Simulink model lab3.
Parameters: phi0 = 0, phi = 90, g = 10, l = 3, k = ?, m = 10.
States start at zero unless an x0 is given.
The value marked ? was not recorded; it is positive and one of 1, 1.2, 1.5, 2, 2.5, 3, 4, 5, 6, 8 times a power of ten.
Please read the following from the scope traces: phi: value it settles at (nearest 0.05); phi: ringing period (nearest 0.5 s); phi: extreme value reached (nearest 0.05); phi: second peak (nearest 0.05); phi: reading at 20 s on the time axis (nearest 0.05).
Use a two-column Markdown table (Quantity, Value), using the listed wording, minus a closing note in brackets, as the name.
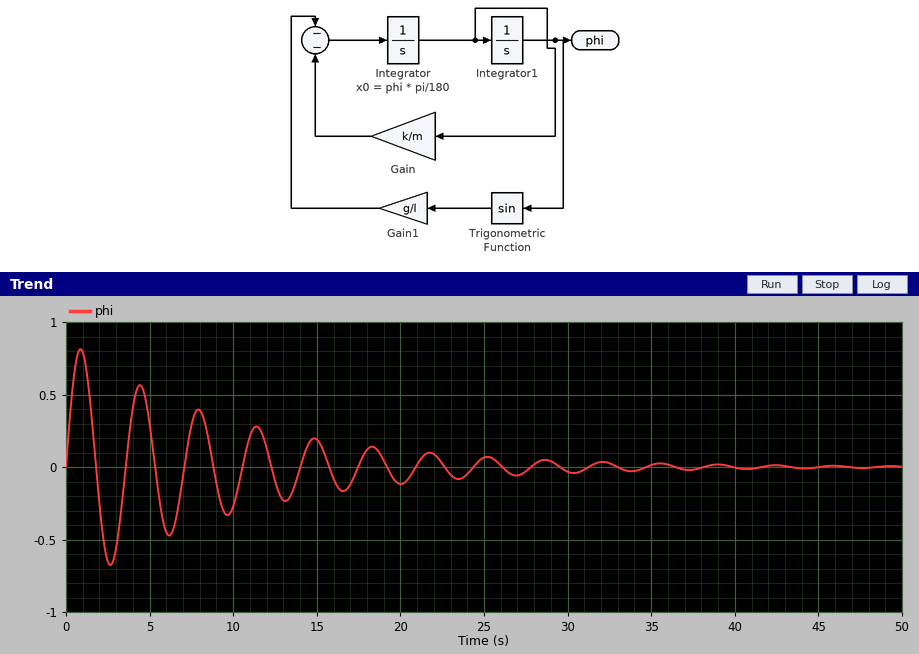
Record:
| Quantity | Value |
|---|---|
| phi: value it settles at | 0.00 |
| phi: ringing period | 3.5 s |
| phi: extreme value reached | 0.80 |
| phi: second peak | 0.55 |
| phi: reading at 20 s on the time axis | -0.10 |
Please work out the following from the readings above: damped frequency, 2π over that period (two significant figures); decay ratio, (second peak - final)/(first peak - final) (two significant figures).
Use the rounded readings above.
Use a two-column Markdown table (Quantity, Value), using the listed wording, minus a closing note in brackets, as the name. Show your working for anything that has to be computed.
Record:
| Quantity | Value |
|---|---|
| damped frequency, 2π over that period | 2π / 3.5 = 1.8 rad/s |
| decay ratio, (second peak - final)/(first peak - final) | (0.55 - 0) / (0.8 - 0) = 0.69 |
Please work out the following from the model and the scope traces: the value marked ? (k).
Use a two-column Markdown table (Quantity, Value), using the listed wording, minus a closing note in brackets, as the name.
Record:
| Quantity | Value |
|---|---|
| the value marked ? | 2 |
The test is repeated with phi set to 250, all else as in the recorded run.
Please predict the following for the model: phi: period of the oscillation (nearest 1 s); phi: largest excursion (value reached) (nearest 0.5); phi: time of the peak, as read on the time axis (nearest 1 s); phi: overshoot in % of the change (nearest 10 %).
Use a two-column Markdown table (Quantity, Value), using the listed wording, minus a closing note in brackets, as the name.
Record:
| Quantity | Value |
|---|---|
| phi: period of the oscillation | 4 s |
| phi: largest excursion (value reached) | 8.5 |
| phi: time of the peak, as read on the time axis | 4 s |
| phi: overshoot in % of the change | 30 % |
